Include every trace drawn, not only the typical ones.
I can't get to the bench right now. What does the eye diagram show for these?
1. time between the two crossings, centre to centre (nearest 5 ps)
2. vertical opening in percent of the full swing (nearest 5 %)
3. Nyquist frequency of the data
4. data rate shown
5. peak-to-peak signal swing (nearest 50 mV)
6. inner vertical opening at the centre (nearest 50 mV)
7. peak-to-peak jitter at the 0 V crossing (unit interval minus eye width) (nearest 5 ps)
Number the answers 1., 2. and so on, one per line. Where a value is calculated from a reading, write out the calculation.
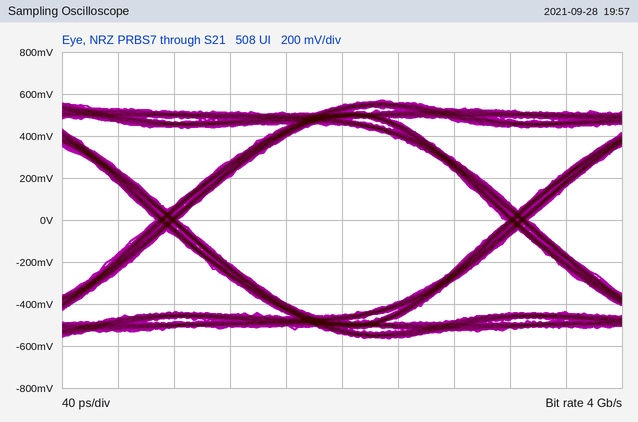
1. 250 ps
2. 900 mV / 1.15 V ≈ 78.3 %, so 80 % to the nearest 5 %
3. 2 GHz
4. 4 Gb/s
5. 1.15 V
6. 900 mV
7. 15 ps
